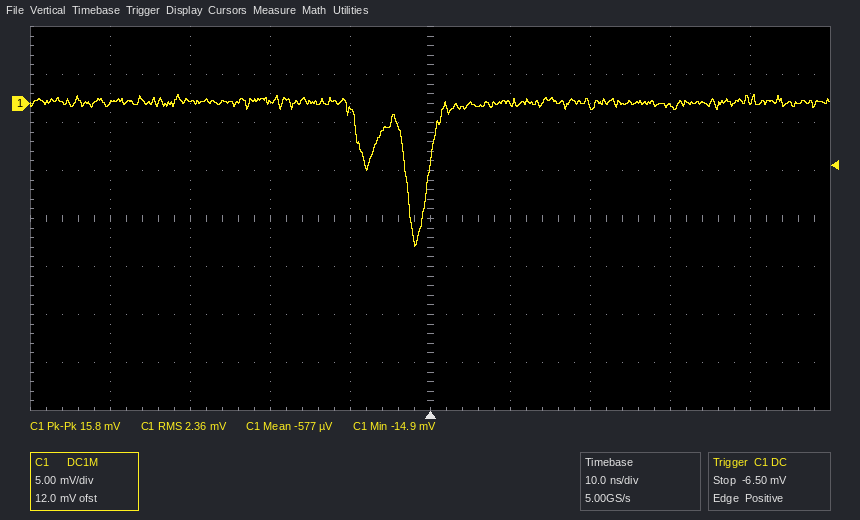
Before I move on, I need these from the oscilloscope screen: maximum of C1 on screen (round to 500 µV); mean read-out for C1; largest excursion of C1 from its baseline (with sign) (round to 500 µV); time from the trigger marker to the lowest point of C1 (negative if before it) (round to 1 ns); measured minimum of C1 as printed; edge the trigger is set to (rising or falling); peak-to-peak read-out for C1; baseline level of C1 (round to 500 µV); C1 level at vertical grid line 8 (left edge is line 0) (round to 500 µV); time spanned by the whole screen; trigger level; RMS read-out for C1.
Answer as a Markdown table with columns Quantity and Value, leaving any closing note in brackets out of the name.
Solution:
| Quantity | Value |
|---|---|
| maximum of C1 on screen | 1.0 mV |
| mean read-out for C1 | -577 µV |
| largest excursion of C1 from its baseline (with sign) | -15.0 mV |
| time from the trigger marker to the lowest point of C1 (negative if before it) | -2 ns |
| measured minimum of C1 as printed | -14.9 mV |
| edge the trigger is set to | rising |
| peak-to-peak read-out for C1 | 15.8 mV |
| baseline level of C1 | 0.0 mV |
| C1 level at vertical grid line 8 (left edge is line 0) | -500 µV |
| time spanned by the whole screen | 100 ns |
| trigger level | -6.50 mV |
| RMS read-out for C1 | 2.36 mV |
